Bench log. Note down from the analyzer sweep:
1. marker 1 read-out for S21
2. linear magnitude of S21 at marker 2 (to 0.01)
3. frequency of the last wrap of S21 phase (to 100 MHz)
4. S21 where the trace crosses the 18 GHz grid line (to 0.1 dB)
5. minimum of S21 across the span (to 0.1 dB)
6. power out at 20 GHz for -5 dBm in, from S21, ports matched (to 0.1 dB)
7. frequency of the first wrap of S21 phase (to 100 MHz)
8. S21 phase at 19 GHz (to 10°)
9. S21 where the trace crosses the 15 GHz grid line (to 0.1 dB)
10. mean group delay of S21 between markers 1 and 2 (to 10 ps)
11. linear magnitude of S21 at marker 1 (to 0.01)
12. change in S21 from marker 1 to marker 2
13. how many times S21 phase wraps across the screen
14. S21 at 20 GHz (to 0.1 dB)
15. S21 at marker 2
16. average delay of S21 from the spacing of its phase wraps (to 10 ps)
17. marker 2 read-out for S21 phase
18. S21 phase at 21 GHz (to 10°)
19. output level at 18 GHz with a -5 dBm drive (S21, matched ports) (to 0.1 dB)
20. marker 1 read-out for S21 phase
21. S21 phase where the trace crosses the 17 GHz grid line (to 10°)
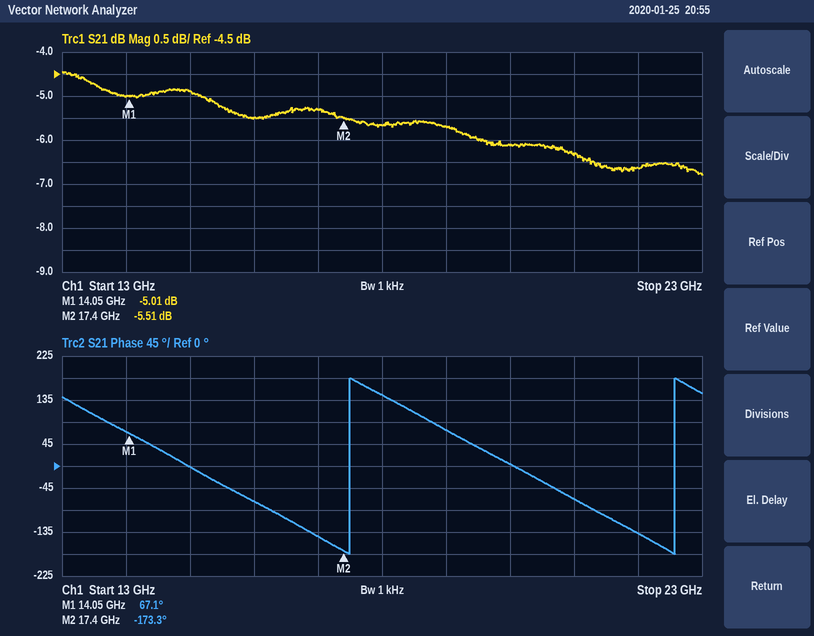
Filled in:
-5.01 dB
0.53
22.6 GHz
-5.7 dB
-6.8 dB
-11.1 dBm
17.5 GHz
70°
-4.9 dB
200 ps
0.56
-0.50 dB
2
-6.1 dB
-5.51 dB
200 ps
-173.3°
-70°
-10.7 dBm
67.1°
-140°
